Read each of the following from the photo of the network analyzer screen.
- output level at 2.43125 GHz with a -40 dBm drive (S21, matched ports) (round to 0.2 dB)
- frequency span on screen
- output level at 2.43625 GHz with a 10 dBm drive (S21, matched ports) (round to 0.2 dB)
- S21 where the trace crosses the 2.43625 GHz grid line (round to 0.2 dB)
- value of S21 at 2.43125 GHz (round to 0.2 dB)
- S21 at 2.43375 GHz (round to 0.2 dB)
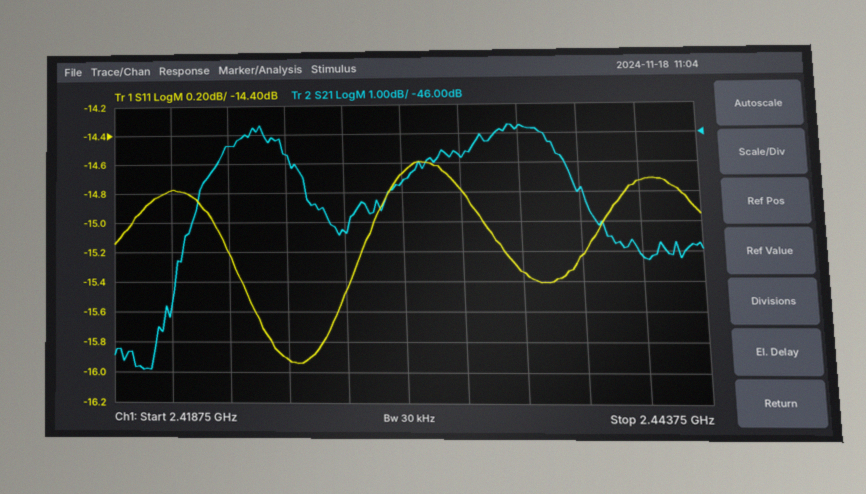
-87.6 dBm
25 MHz
-35.8 dBm
-45.8 dB
-47.6 dB
-46.8 dB
